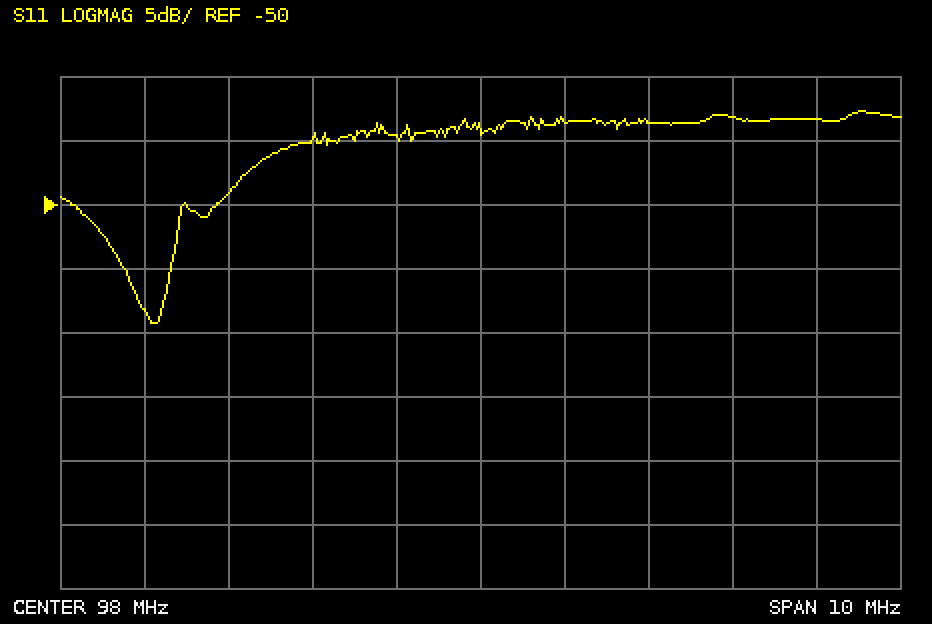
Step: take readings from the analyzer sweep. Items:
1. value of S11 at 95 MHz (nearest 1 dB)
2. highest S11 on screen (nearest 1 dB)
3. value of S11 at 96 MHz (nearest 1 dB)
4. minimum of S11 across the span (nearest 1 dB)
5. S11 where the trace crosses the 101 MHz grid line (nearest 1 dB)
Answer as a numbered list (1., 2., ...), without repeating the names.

1. -49 dB
2. -43 dB
3. -45 dB
4. -59 dB
5. -43 dB
